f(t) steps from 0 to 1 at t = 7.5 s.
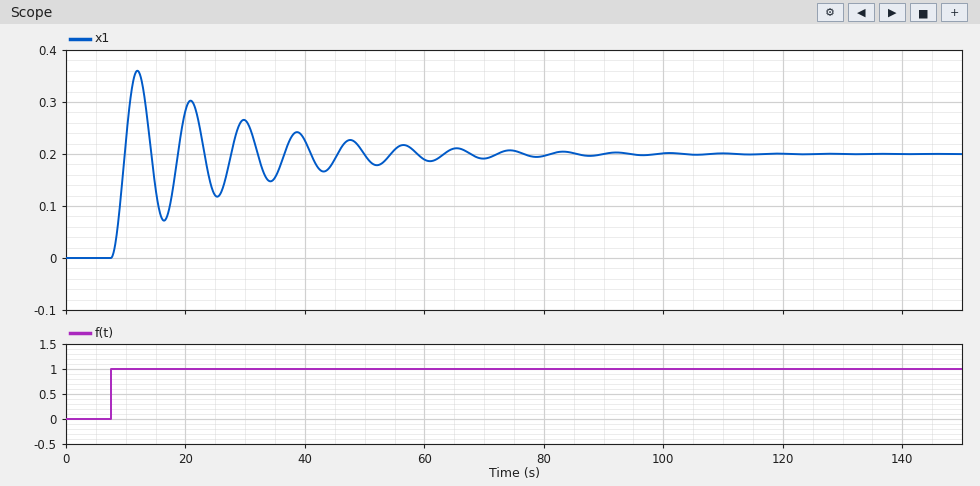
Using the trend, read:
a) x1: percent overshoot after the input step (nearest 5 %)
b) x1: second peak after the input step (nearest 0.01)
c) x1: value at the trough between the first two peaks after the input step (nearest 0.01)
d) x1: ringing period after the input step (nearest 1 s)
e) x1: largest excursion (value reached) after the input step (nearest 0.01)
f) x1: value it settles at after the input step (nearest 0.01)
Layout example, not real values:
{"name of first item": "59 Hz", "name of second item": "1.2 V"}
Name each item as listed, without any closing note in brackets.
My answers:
{"x1: percent overshoot after the input step": "80 %", "x1: second peak after the input step": "0.30", "x1: value at the trough between the first two peaks after the input step": "0.07", "x1: ringing period after the input step": "9 s", "x1: largest excursion (value reached) after the input step": "0.36", "x1: value it settles at after the input step": "0.20"}
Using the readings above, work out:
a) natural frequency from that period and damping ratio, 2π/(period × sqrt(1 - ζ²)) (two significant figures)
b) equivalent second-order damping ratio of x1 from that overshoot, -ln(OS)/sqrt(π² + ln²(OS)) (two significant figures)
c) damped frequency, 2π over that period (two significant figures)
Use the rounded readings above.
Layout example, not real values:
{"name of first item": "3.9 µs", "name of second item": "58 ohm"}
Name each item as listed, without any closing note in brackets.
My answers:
{"natural frequency from that period and damping ratio, 2π/(period × sqrt(1 - ζ²))": "0.70 rad/s", "equivalent second-order damping ratio of x1 from that overshoot, -ln(OS)/sqrt(π² + ln²(OS))": "0.071", "damped frequency, 2π over that period": "0.70 rad/s"}
